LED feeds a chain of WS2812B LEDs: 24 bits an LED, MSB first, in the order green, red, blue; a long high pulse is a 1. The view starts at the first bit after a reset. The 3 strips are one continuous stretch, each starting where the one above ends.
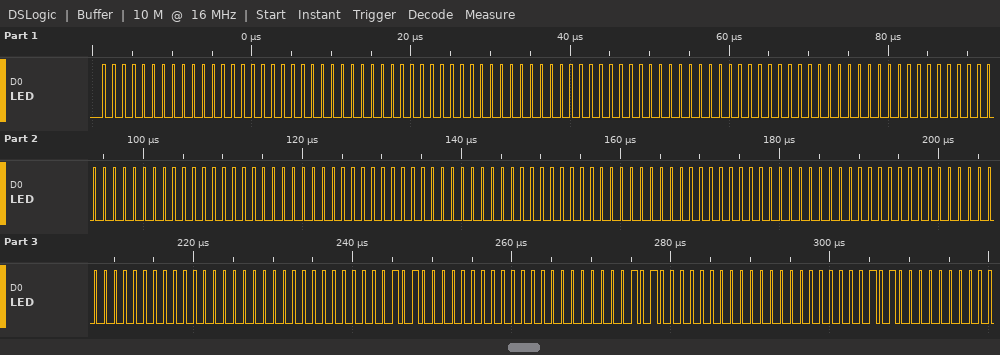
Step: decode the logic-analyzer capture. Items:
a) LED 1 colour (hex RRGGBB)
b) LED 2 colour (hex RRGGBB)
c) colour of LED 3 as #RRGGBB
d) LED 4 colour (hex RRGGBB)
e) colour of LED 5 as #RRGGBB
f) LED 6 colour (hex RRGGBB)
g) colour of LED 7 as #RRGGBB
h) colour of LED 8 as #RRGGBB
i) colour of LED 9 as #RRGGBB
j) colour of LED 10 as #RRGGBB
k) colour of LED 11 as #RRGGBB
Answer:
#000000
#000000
#000000
#000000
#000000
#000000
#000000
#000000
#000014
#000014
#000014
